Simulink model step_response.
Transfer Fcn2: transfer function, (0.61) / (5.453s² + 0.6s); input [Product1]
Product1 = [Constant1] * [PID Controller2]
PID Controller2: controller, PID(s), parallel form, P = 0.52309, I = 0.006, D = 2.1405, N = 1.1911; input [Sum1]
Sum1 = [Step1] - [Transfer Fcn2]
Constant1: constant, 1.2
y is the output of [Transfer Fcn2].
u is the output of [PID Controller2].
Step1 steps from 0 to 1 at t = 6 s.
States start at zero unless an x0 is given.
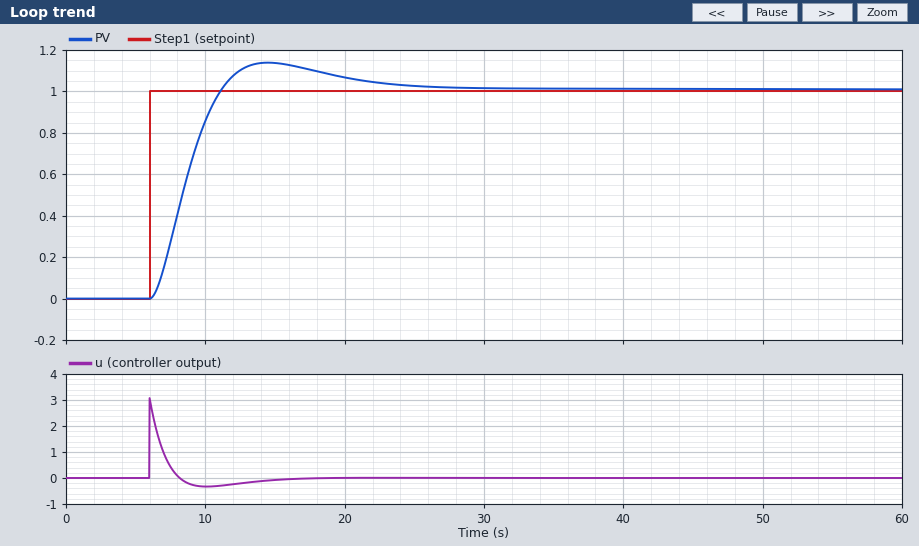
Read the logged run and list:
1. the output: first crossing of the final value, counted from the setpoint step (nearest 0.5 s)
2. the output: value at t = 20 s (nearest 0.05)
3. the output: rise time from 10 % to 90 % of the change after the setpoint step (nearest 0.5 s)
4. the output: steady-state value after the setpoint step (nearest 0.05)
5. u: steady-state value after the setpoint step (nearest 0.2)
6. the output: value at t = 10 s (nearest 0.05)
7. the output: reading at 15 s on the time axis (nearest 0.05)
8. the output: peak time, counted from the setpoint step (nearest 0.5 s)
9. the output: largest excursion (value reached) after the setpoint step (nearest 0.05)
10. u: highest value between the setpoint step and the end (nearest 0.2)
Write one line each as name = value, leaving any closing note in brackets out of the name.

the output: first crossing of the final value, counted from the setpoint step = 5.0 s
the output: value at t = 20 s = 1.05
the output: rise time from 10 % to 90 % of the change after the setpoint step = 3.5 s
the output: steady-state value after the setpoint step = 1.00
u: steady-state value after the setpoint step = 0.0
the output: value at t = 10 s = 0.85
the output: reading at 15 s on the time axis = 1.15
the output: peak time, counted from the setpoint step = 8.5 s
the output: largest excursion (value reached) after the setpoint step = 1.15
u: highest value between the setpoint step and the end = 3.0
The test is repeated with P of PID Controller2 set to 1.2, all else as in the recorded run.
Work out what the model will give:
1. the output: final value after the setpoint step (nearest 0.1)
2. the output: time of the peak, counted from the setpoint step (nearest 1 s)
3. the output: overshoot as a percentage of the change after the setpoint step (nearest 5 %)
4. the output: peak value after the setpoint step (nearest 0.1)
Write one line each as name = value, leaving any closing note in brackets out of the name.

the output: final value after the setpoint step = 1.0
the output: time of the peak, counted from the setpoint step = 6 s
the output: overshoot as a percentage of the change after the setpoint step = 30 %
the output: peak value after the setpoint step = 1.3
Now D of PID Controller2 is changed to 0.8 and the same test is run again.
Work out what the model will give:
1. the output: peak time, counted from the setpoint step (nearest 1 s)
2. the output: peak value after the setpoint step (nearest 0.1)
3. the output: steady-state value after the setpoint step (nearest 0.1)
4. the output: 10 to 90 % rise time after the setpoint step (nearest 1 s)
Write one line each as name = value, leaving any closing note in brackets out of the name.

the output: peak time, counted from the setpoint step = 11 s
the output: peak value after the setpoint step = 1.3
the output: steady-state value after the setpoint step = 1.0
the output: 10 to 90 % rise time after the setpoint step = 4 s
